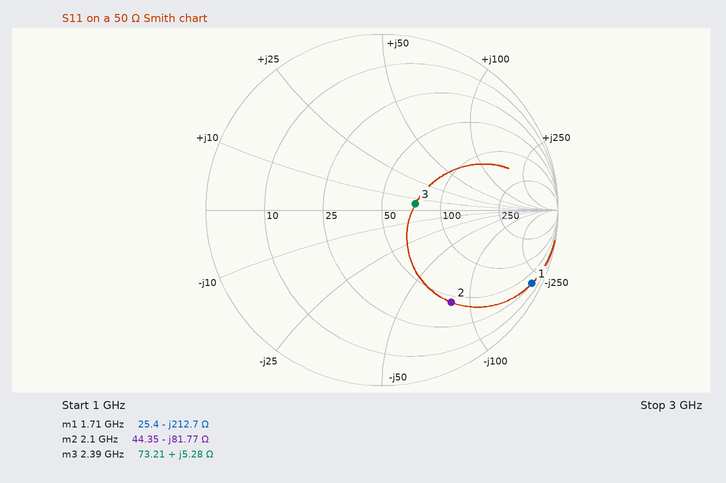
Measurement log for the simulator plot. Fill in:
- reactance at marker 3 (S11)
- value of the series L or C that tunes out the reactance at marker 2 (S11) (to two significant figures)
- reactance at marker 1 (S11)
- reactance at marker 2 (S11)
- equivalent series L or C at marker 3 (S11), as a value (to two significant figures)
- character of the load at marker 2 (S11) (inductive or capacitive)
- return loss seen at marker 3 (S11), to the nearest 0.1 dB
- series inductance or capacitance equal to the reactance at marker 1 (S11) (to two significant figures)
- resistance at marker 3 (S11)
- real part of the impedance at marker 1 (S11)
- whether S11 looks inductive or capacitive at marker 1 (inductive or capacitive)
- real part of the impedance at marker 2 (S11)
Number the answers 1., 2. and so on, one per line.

1. +5.28 Ω
2. 6.2 nH
3. -212.7 Ω
4. -81.77 Ω
5. 350 pH
6. capacitive
7. 14.3 dB
8. 440 fF
9. 73.21 Ω
10. 25.4 Ω
11. capacitive
12. 44.35 Ω
